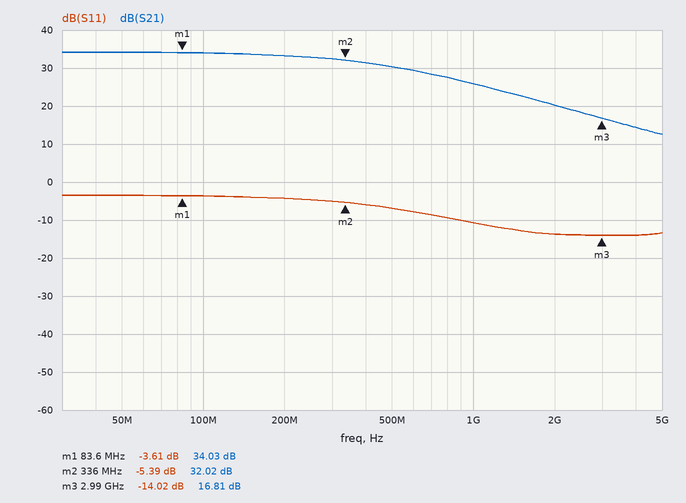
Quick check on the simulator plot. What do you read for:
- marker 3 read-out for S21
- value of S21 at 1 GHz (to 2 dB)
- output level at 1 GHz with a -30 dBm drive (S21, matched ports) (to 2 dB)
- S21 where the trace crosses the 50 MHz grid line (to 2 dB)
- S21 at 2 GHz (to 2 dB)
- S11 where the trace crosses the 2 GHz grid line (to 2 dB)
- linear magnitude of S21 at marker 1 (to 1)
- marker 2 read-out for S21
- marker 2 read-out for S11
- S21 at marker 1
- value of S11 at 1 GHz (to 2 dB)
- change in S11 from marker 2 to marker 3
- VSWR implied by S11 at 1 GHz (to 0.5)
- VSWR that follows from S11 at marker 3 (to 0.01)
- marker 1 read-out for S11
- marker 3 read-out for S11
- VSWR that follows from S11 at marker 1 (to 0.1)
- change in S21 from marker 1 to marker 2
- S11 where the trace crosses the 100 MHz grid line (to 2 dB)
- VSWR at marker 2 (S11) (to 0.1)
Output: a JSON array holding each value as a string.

["16.81 dB", "26 dB", "-4 dBm", "34 dB", "20 dB", "-14 dB", "50", "32.02 dB", "-5.39 dB", "34.03 dB", "-10 dB", "-8.63 dB", "2.0", "1.50", "-3.61 dB", "-14.02 dB", "4.9", "-2.01 dB", "-4 dB", "3.3"]
